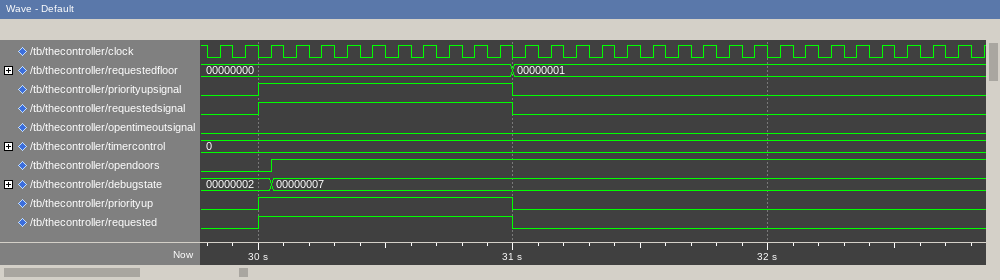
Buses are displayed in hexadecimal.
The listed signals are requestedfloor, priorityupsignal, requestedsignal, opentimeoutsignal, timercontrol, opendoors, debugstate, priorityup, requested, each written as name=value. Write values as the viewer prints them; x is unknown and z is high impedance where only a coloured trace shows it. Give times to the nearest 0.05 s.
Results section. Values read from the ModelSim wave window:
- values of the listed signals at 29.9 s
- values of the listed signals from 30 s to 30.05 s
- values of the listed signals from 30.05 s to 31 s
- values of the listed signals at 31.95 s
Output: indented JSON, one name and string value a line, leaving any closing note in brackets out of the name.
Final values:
{
  "values of the listed signals at 29.9 s": "requestedfloor=00000000, priorityupsignal=0, requestedsignal=0, opentimeoutsignal=0, timercontrol=0, opendoors=0, debugstate=00000002, priorityup=0, requested=0",
  "values of the listed signals from 30 s to 30.05 s": "requestedfloor=00000000, priorityupsignal=1, requestedsignal=1, opentimeoutsignal=0, timercontrol=0, opendoors=0, debugstate=00000002, priorityup=1, requested=1",
  "values of the listed signals from 30.05 s to 31 s": "requestedfloor=00000000, priorityupsignal=1, requestedsignal=1, opentimeoutsignal=0, timercontrol=0, opendoors=1, debugstate=00000007, priorityup=1, requested=1",
  "values of the listed signals at 31.95 s": "requestedfloor=00000001, priorityupsignal=0, requestedsignal=0, opentimeoutsignal=0, timercontrol=0, opendoors=1, debugstate=00000007, priorityup=0, requested=0"
}
